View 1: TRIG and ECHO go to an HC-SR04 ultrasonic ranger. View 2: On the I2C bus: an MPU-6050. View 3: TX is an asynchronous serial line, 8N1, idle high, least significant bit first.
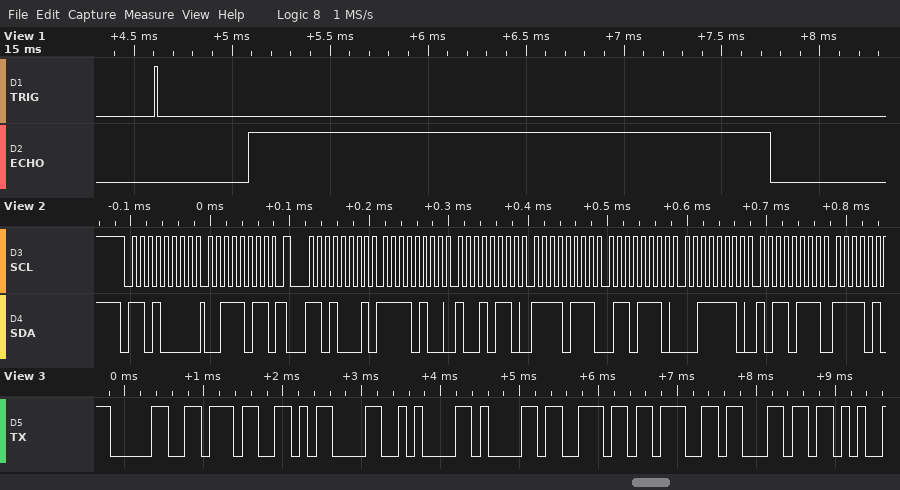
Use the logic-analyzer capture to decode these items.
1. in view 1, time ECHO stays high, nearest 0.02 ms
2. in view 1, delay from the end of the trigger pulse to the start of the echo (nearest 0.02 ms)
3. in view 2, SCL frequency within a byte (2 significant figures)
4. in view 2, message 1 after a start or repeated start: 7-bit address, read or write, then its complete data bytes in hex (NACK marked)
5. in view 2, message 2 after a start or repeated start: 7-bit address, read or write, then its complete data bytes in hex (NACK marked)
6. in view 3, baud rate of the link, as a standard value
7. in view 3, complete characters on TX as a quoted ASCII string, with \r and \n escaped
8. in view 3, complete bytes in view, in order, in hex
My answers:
2.66 ms
0.46 ms
100 kHz
0x68 write: 3B
0x68 read: F4 96 F7 6E 3E B7
9600 baud
"07\r\nangl"
30 37 0D 0A 61 6E 67 6C
